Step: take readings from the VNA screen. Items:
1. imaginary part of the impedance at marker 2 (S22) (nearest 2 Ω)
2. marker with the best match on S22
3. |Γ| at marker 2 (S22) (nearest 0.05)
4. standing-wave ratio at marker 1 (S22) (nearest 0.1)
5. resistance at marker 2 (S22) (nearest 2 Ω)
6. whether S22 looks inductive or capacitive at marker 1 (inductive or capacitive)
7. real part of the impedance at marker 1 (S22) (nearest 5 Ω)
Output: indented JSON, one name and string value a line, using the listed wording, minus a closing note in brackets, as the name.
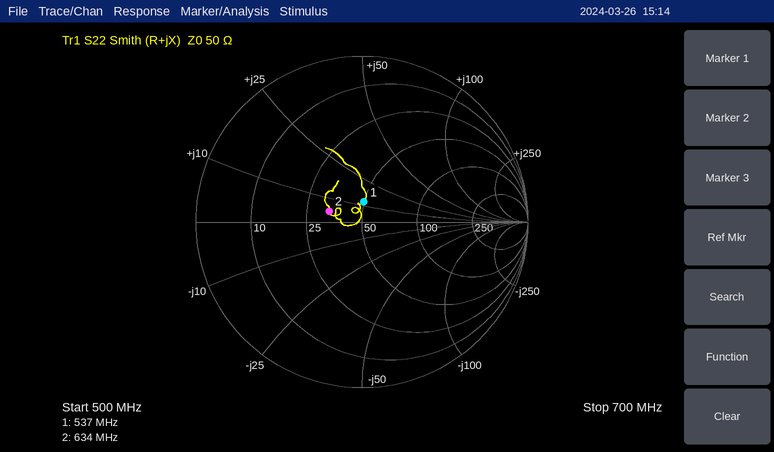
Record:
{
  "imaginary part of the impedance at marker 2 (S22)": "+4 Ω",
  "marker with the best match on S22": "marker 1",
  "|Γ| at marker 2 (S22)": "0.20",
  "standing-wave ratio at marker 1 (S22)": "1.3",
  "resistance at marker 2 (S22)": "34 Ω",
  "whether S22 looks inductive or capacitive at marker 1": "inductive",
  "real part of the impedance at marker 1 (S22)": "50 Ω"
}
